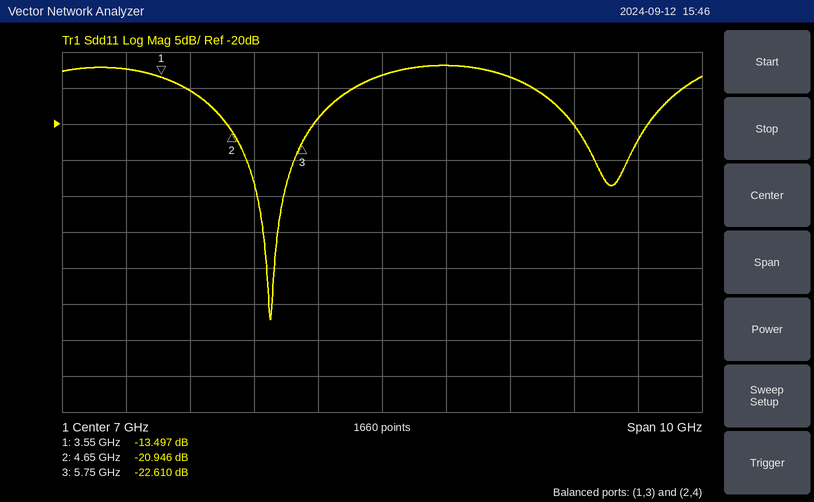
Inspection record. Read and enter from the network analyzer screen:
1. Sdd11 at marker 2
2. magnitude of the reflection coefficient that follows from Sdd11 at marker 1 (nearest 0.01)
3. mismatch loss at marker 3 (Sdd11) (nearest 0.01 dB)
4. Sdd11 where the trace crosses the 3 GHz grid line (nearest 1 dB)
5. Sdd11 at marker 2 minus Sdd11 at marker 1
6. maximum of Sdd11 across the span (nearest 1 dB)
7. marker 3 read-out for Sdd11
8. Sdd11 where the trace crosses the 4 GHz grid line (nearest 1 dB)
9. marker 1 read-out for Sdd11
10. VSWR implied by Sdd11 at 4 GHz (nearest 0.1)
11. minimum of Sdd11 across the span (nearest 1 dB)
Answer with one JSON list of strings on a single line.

["-20.946 dB", "0.21", "0.02 dB", "-12 dB", "-7.449 dB", "-12 dB", "-22.610 dB", "-15 dB", "-13.497 dB", "1.4", "-47 dB"]
